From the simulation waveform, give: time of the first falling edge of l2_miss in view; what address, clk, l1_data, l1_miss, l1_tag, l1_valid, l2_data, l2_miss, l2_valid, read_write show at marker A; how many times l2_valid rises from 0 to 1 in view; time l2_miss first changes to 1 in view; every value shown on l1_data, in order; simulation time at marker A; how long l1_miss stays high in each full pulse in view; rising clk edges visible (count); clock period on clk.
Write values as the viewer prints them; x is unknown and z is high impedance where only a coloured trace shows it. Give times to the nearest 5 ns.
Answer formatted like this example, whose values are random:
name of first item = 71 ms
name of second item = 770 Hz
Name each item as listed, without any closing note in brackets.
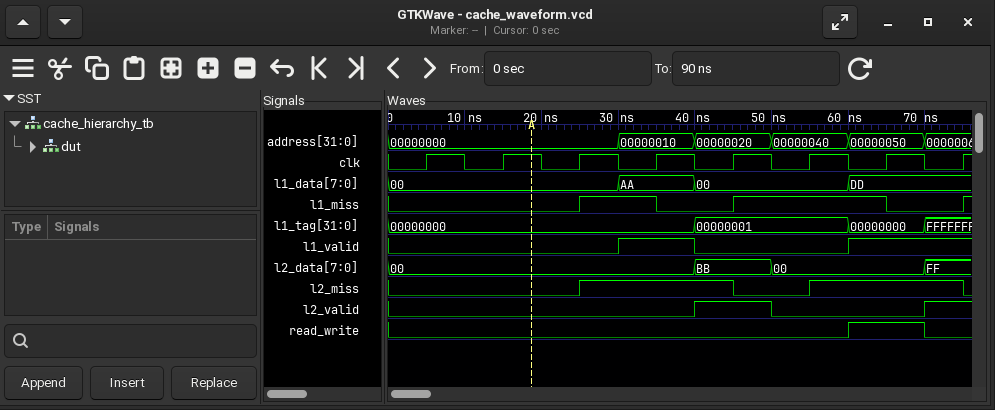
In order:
time of the first falling edge of l2_miss in view = 45 ns
what address, clk, l1_data, l1_miss, l1_tag, l1_valid, l2_data, l2_miss, l2_valid, read_write show at marker A = address=00000000, clk=1, l1_data=00, l1_miss=0, l1_tag=00000000, l1_valid=0, l2_data=00, l2_miss=0, l2_valid=0, read_write=0
how many times l2_valid rises from 0 to 1 in view = 2
time l2_miss first changes to 1 in view = 25 ns
every value shown on l1_data, in order = 00, AA, 00, DD
simulation time at marker A = 20 ns
how long l1_miss stays high in each full pulse in view = 10 ns, 20 ns
rising clk edges visible = 8
clock period on clk = 10 ns
